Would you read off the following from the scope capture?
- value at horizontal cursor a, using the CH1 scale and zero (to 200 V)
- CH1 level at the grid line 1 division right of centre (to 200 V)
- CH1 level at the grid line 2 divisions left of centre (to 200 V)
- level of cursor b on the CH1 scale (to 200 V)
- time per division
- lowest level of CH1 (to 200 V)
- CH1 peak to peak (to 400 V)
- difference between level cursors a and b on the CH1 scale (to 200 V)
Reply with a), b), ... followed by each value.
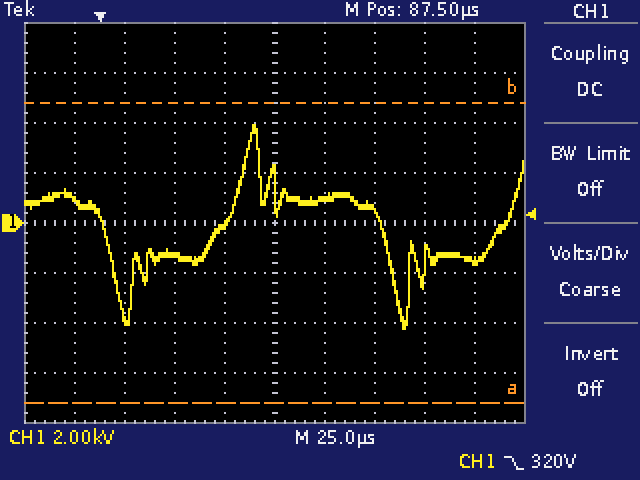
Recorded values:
a) -7.2 kV
b) 1.0 kV
c) -1.2 kV
d) 4.8 kV
e) 25 µs
f) -4.2 kV
g) 8.0 kV
h) 12.0 kV
